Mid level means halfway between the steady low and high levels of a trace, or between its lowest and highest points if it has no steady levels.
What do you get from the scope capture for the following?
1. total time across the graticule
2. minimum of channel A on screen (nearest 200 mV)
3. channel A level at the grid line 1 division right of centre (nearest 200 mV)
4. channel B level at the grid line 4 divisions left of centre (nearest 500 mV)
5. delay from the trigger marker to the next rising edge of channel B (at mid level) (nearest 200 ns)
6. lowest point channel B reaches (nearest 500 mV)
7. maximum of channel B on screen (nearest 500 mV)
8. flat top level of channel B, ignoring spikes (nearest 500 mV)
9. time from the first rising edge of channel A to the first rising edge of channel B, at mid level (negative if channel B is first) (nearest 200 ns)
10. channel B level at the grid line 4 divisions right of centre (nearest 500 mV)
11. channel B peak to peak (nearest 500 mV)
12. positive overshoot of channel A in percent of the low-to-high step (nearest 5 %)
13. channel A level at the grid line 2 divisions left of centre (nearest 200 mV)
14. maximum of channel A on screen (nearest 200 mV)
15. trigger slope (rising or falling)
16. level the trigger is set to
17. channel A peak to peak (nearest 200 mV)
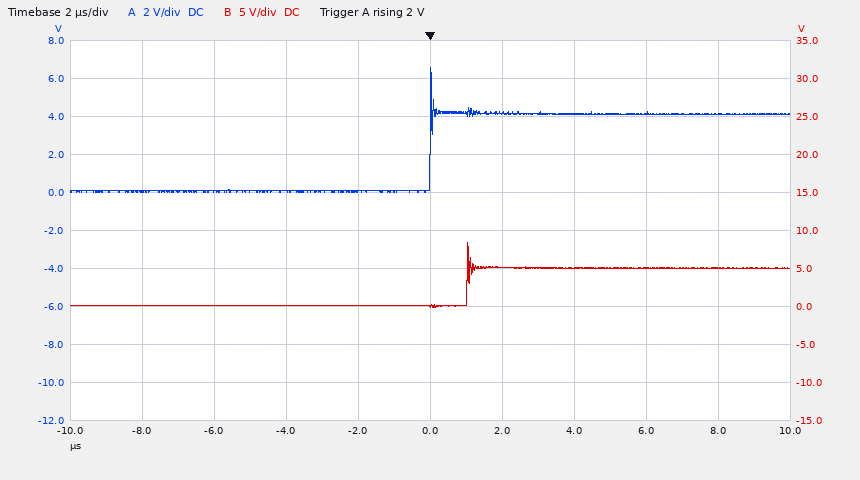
20 µs
0.0 V
4.2 V
0.0 V
1.0 µs
0.0 V
8.5 V
5.0 V
+1.0 µs
5.0 V
8.5 V
60 %
0.0 V
6.6 V
rising
2 V
6.6 V
